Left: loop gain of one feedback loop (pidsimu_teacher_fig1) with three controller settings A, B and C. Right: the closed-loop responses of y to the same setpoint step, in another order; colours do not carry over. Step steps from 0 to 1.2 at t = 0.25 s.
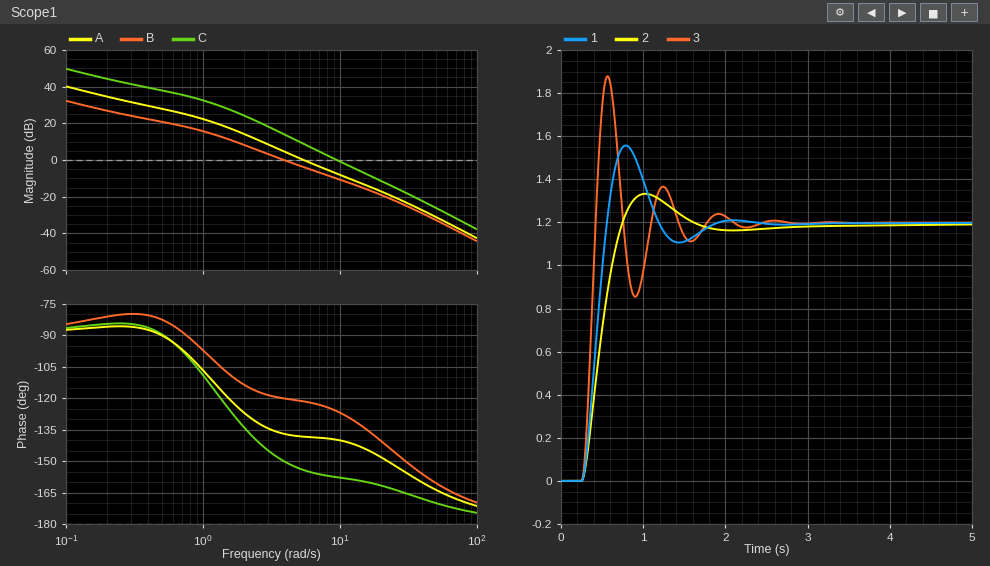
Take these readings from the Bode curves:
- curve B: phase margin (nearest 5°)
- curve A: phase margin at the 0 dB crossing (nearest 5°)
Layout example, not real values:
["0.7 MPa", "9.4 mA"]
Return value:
["60°", "40°"]
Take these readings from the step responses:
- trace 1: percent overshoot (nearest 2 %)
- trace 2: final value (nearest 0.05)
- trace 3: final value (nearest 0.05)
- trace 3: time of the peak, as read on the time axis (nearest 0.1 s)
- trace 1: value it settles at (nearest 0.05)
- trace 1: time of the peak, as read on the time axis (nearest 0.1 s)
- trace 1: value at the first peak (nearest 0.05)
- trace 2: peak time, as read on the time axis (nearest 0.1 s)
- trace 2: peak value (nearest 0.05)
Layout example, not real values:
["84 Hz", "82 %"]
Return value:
["30 %", "1.20", "1.20", "0.6 s", "1.20", "0.8 s", "1.55", "1.0 s", "1.35"]
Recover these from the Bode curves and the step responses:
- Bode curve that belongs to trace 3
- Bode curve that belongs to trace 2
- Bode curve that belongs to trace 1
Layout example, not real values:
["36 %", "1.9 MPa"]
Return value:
["C", "B", "A"]
